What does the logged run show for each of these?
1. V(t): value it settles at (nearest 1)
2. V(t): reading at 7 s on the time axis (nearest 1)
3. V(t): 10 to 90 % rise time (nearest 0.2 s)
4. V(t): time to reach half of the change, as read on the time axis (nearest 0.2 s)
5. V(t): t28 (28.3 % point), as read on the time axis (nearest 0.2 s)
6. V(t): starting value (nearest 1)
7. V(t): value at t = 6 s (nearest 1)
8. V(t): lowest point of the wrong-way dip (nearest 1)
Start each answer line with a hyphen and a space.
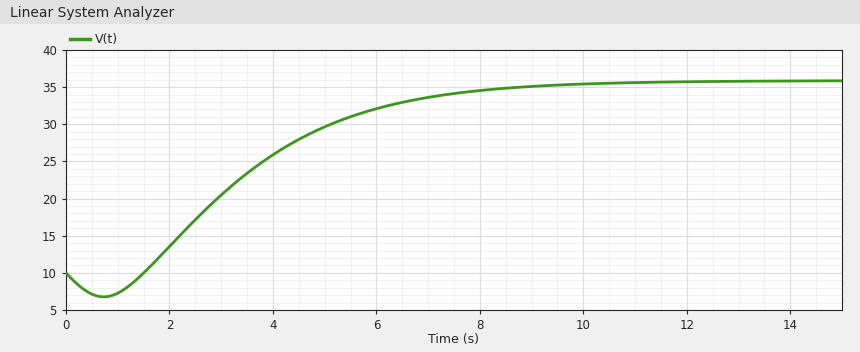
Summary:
- 36
- 34
- 4.8 s
- 3.4 s
- 2.6 s
- 10
- 32
- 7
